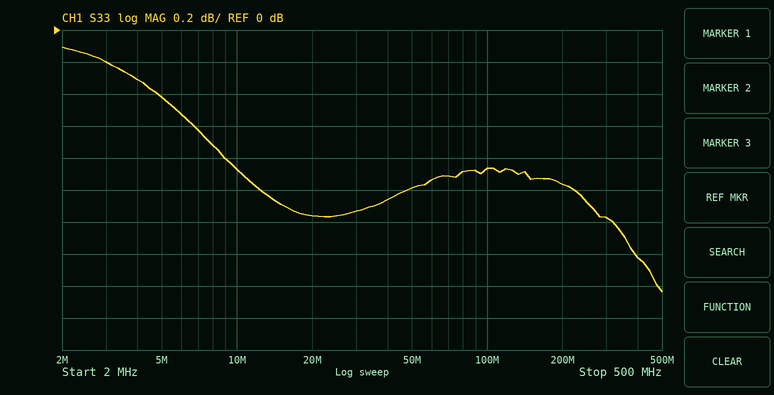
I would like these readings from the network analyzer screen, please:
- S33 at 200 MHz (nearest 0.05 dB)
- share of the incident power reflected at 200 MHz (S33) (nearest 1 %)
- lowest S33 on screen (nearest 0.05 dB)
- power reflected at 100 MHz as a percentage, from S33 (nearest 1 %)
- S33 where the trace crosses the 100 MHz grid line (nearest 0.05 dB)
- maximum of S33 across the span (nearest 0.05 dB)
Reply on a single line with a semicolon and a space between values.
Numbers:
-0.95 dB; 80 %; -1.65 dB; 82 %; -0.85 dB; -0.10 dB
